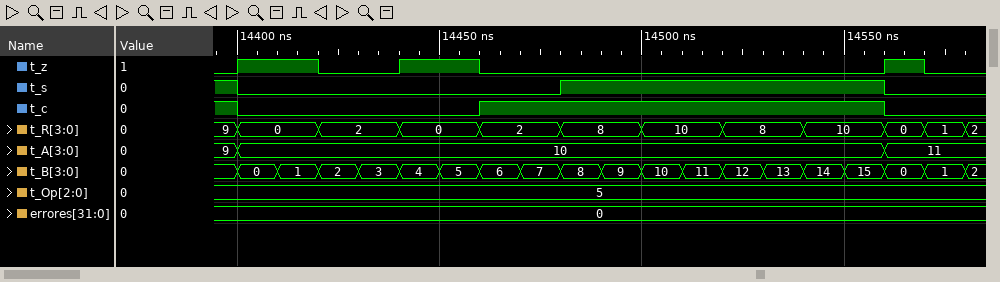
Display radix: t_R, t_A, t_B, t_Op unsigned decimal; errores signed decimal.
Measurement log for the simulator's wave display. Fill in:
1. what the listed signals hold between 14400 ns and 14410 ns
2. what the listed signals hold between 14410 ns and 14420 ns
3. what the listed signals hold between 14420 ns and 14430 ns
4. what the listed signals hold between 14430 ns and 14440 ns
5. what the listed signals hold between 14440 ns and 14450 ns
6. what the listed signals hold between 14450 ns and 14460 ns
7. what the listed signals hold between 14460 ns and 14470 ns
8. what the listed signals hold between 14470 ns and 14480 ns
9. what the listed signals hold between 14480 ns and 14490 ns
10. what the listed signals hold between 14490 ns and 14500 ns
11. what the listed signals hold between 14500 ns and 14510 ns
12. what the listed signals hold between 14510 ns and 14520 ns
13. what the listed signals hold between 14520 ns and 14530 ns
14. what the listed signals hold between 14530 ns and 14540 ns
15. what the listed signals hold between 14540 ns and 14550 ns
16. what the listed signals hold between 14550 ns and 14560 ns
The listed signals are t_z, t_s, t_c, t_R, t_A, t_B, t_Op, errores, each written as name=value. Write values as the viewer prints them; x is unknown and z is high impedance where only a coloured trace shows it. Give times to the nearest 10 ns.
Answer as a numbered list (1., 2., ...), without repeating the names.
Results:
1. t_z=1, t_s=0, t_c=0, t_R=0, t_A=10, t_B=0, t_Op=5, errores=0
2. t_z=1, t_s=0, t_c=0, t_R=0, t_A=10, t_B=1, t_Op=5, errores=0
3. t_z=0, t_s=0, t_c=0, t_R=2, t_A=10, t_B=2, t_Op=5, errores=0
4. t_z=0, t_s=0, t_c=0, t_R=2, t_A=10, t_B=3, t_Op=5, errores=0
5. t_z=1, t_s=0, t_c=0, t_R=0, t_A=10, t_B=4, t_Op=5, errores=0
6. t_z=1, t_s=0, t_c=0, t_R=0, t_A=10, t_B=5, t_Op=5, errores=0
7. t_z=0, t_s=0, t_c=1, t_R=2, t_A=10, t_B=6, t_Op=5, errores=0
8. t_z=0, t_s=0, t_c=1, t_R=2, t_A=10, t_B=7, t_Op=5, errores=0
9. t_z=0, t_s=1, t_c=1, t_R=8, t_A=10, t_B=8, t_Op=5, errores=0
10. t_z=0, t_s=1, t_c=1, t_R=8, t_A=10, t_B=9, t_Op=5, errores=0
11. t_z=0, t_s=1, t_c=1, t_R=10, t_A=10, t_B=10, t_Op=5, errores=0
12. t_z=0, t_s=1, t_c=1, t_R=10, t_A=10, t_B=11, t_Op=5, errores=0
13. t_z=0, t_s=1, t_c=1, t_R=8, t_A=10, t_B=12, t_Op=5, errores=0
14. t_z=0, t_s=1, t_c=1, t_R=8, t_A=10, t_B=13, t_Op=5, errores=0
15. t_z=0, t_s=1, t_c=1, t_R=10, t_A=10, t_B=14, t_Op=5, errores=0
16. t_z=0, t_s=1, t_c=1, t_R=10, t_A=10, t_B=15, t_Op=5, errores=0
